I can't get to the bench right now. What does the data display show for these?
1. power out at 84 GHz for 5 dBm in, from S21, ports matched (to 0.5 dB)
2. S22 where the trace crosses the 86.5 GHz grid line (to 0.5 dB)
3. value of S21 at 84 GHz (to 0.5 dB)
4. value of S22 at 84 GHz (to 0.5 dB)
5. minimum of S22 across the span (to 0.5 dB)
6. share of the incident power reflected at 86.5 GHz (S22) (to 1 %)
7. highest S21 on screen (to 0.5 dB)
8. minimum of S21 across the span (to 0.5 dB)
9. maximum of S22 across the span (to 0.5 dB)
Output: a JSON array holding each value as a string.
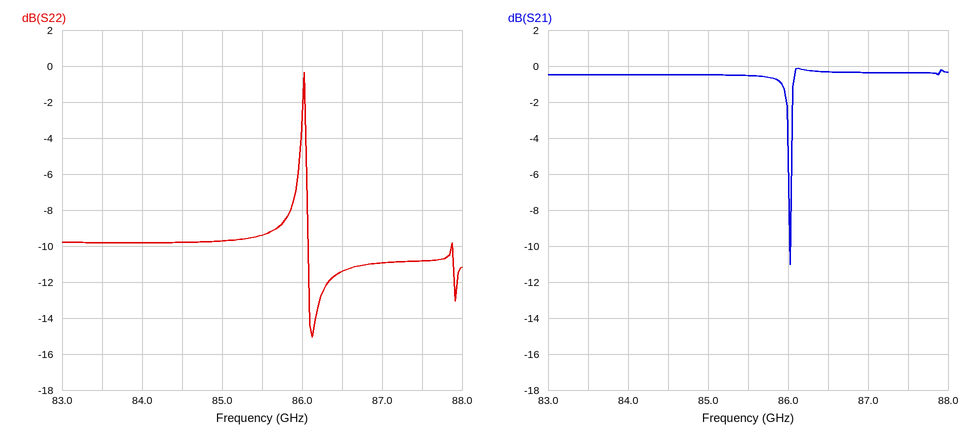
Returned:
["4.5 dBm", "-11.5 dB", "-0.5 dB", "-10.0 dB", "-15.0 dB", "7 %", "0.0 dB", "-11.0 dB", "-0.5 dB"]
